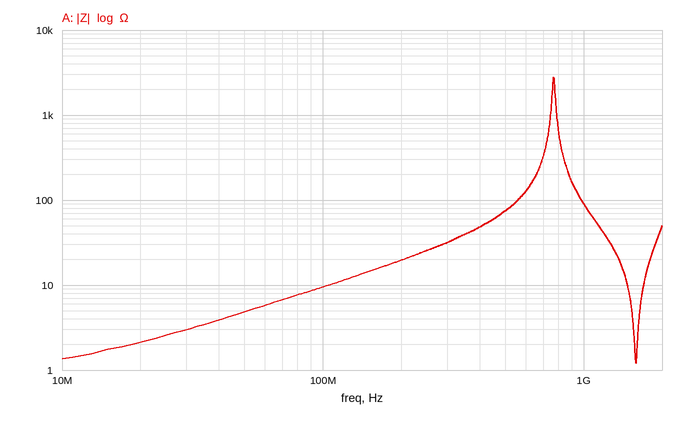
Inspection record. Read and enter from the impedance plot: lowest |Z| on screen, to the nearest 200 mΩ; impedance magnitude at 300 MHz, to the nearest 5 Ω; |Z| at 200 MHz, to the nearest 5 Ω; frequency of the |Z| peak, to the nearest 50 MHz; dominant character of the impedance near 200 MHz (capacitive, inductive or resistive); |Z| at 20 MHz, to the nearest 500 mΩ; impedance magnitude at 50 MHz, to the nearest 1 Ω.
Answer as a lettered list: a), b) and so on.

a) 1.2 Ω
b) 30 Ω
c) 20 Ω
d) 750 MHz
e) inductive
f) 2.0 Ω
g) 5 Ω
